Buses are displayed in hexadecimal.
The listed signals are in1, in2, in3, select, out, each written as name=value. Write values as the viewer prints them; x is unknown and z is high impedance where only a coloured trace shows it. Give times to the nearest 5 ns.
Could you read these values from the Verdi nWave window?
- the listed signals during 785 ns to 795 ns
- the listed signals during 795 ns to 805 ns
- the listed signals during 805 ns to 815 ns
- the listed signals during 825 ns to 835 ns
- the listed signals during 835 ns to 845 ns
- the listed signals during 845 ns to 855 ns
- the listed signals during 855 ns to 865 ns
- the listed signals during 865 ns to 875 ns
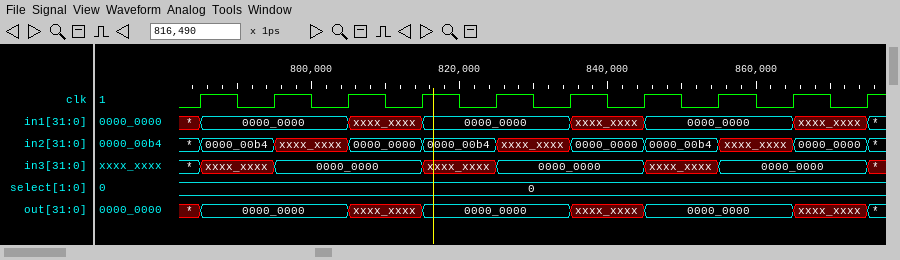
in1=0000_0000, in2=0000_00b4, in3=xxxx_xxxx, select=0, out=0000_0000
in1=0000_0000, in2=xxxx_xxxx, in3=0000_0000, select=0, out=0000_0000
in1=xxxx_xxxx, in2=0000_0000, in3=0000_0000, select=0, out=xxxx_xxxx
in1=0000_0000, in2=xxxx_xxxx, in3=0000_0000, select=0, out=0000_0000
in1=xxxx_xxxx, in2=0000_0000, in3=0000_0000, select=0, out=xxxx_xxxx
in1=0000_0000, in2=0000_00b4, in3=xxxx_xxxx, select=0, out=0000_0000
in1=0000_0000, in2=xxxx_xxxx, in3=0000_0000, select=0, out=0000_0000
in1=xxxx_xxxx, in2=0000_0000, in3=0000_0000, select=0, out=xxxx_xxxx
